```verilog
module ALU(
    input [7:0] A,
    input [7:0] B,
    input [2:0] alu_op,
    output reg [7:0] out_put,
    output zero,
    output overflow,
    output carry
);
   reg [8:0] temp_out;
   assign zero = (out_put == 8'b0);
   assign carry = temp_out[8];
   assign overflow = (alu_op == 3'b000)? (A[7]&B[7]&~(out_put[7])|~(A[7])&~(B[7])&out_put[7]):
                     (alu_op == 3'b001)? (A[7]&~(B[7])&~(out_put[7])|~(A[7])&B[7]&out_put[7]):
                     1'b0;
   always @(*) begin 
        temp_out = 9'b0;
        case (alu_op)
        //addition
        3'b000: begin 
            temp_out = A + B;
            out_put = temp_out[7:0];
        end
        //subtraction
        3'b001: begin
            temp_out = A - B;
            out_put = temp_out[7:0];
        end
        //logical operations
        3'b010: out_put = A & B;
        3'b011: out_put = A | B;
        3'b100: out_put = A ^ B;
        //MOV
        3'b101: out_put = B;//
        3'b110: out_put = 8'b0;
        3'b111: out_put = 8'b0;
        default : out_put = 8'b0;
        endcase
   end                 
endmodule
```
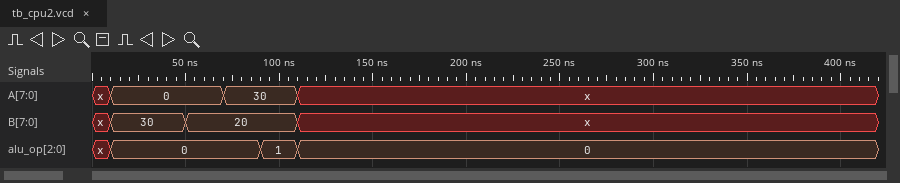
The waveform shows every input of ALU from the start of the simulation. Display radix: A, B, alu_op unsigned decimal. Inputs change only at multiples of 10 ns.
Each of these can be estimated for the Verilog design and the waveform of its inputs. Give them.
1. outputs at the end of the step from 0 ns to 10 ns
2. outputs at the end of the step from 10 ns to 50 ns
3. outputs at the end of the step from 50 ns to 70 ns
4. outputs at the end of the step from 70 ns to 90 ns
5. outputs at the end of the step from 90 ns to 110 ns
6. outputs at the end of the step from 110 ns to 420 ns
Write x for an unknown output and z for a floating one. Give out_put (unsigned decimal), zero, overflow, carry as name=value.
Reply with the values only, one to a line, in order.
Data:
out_put=x, zero=x, overflow=x, carry=x
out_put=30, zero=0, overflow=0, carry=0
out_put=20, zero=0, overflow=0, carry=0
out_put=50, zero=0, overflow=0, carry=0
out_put=10, zero=0, overflow=0, carry=0
out_put=x, zero=x, overflow=x, carry=x
